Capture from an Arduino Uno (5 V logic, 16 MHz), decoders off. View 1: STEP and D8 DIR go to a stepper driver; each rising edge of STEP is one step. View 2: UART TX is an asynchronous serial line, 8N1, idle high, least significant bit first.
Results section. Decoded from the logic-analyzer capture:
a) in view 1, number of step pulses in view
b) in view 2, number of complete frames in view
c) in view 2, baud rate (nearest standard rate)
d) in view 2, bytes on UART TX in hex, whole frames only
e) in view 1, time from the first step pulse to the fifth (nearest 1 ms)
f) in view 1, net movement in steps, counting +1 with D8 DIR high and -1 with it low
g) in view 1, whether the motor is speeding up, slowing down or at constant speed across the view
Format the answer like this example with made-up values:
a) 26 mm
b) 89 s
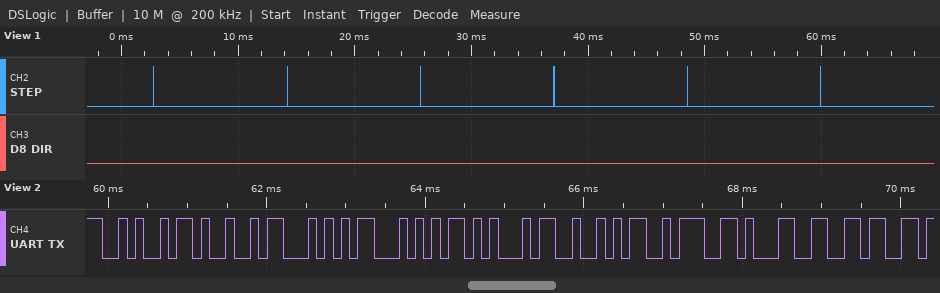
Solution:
a) 6
b) 9
c) 9600 baud
d) 0x4A 0x49 0x54 0x54 0x45 0x52 0x3A 0x31 0x36
e) 46 ms
f) -6
g) constant speed
